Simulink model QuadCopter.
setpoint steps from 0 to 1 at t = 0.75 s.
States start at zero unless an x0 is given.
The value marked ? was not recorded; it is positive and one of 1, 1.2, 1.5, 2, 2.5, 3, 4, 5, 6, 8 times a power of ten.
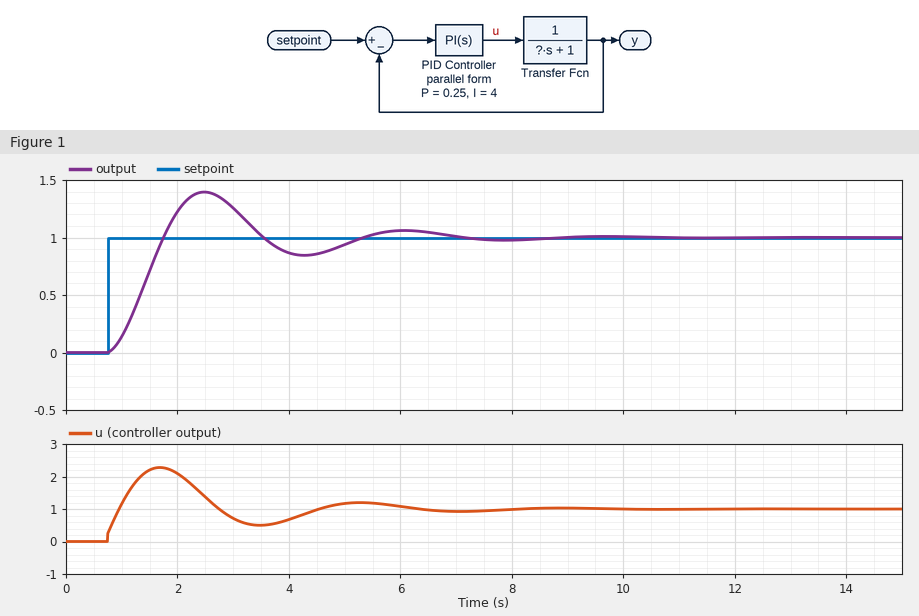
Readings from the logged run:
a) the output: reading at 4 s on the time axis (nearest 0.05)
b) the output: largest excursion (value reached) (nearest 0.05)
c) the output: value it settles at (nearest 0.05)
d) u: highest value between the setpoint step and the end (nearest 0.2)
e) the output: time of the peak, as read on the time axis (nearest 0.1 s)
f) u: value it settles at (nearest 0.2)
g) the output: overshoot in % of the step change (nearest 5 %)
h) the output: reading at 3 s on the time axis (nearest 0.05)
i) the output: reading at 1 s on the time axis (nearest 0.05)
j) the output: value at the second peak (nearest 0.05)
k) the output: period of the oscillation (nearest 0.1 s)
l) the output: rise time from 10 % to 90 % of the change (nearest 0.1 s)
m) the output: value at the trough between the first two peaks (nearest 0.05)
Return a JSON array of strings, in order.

["0.85", "1.40", "1.00", "2.2", "2.5 s", "1.0", "40 %", "1.25", "0.15", "1.05", "3.6 s", "0.7 s", "0.85"]
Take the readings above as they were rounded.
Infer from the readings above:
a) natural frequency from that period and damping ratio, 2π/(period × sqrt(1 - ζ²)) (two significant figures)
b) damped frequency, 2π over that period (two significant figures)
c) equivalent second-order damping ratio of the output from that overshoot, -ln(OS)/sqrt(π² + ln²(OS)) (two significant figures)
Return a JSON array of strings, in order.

["1.8 rad/s", "1.7 rad/s", "0.28"]
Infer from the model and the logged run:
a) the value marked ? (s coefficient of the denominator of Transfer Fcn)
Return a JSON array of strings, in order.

["1.2"]
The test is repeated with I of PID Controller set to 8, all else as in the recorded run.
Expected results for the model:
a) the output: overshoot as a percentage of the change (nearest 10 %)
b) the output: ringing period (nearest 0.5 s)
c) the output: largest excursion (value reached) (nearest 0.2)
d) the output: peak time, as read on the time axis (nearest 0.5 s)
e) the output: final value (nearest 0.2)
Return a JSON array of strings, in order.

["50 %", "2.5 s", "1.6", "2.0 s", "1.0"]
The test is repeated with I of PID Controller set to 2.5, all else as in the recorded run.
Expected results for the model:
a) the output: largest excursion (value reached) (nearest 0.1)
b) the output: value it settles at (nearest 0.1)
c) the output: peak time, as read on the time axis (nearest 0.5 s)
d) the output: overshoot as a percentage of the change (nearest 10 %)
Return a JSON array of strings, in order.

["1.3", "1.0", "3.0 s", "30 %"]
